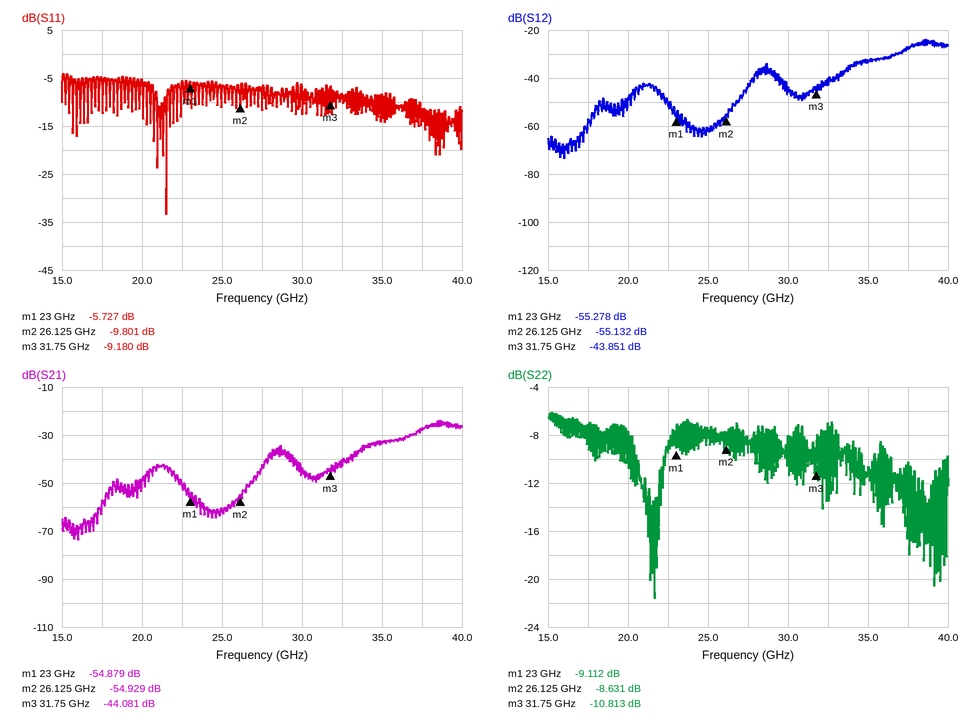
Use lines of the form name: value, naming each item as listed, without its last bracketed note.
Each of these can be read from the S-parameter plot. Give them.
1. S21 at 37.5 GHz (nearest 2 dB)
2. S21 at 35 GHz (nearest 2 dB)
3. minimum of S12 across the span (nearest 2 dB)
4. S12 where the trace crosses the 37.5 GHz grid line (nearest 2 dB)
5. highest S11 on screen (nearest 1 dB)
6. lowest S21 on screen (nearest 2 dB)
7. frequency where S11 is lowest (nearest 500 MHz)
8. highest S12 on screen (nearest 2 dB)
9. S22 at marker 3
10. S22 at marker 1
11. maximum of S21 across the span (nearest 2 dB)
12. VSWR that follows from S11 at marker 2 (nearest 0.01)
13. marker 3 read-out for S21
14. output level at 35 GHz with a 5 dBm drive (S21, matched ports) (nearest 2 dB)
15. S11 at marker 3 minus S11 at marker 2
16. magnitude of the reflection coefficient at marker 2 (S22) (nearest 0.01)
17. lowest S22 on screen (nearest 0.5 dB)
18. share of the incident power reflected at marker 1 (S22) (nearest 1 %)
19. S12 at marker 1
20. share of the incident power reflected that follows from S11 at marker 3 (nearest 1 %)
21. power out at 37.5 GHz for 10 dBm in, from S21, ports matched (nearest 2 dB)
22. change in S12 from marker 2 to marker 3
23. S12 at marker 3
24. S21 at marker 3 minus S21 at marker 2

S21 at 37.5 GHz: -28 dB
S21 at 35 GHz: -34 dB
minimum of S12 across the span: -74 dB
S12 where the trace crosses the 37.5 GHz grid line: -28 dB
highest S11 on screen: -4 dB
lowest S21 on screen: -74 dB
frequency where S11 is lowest: 21.5 GHz
highest S12 on screen: -24 dB
S22 at marker 3: -10.813 dB
S22 at marker 1: -9.112 dB
maximum of S21 across the span: -24 dB
VSWR that follows from S11 at marker 2: 1.96
marker 3 read-out for S21: -44.081 dB
output level at 35 GHz with a 5 dBm drive (S21, matched ports): -28 dBm
S11 at marker 3 minus S11 at marker 2: 0.621 dB
magnitude of the reflection coefficient at marker 2 (S22): 0.37
lowest S22 on screen: -21.5 dB
share of the incident power reflected at marker 1 (S22): 12 %
S12 at marker 1: -55.278 dB
share of the incident power reflected that follows from S11 at marker 3: 12 %
power out at 37.5 GHz for 10 dBm in, from S21, ports matched: -18 dBm
change in S12 from marker 2 to marker 3: 11.281 dB
S12 at marker 3: -43.851 dB
S21 at marker 3 minus S21 at marker 2: 10.848 dB
